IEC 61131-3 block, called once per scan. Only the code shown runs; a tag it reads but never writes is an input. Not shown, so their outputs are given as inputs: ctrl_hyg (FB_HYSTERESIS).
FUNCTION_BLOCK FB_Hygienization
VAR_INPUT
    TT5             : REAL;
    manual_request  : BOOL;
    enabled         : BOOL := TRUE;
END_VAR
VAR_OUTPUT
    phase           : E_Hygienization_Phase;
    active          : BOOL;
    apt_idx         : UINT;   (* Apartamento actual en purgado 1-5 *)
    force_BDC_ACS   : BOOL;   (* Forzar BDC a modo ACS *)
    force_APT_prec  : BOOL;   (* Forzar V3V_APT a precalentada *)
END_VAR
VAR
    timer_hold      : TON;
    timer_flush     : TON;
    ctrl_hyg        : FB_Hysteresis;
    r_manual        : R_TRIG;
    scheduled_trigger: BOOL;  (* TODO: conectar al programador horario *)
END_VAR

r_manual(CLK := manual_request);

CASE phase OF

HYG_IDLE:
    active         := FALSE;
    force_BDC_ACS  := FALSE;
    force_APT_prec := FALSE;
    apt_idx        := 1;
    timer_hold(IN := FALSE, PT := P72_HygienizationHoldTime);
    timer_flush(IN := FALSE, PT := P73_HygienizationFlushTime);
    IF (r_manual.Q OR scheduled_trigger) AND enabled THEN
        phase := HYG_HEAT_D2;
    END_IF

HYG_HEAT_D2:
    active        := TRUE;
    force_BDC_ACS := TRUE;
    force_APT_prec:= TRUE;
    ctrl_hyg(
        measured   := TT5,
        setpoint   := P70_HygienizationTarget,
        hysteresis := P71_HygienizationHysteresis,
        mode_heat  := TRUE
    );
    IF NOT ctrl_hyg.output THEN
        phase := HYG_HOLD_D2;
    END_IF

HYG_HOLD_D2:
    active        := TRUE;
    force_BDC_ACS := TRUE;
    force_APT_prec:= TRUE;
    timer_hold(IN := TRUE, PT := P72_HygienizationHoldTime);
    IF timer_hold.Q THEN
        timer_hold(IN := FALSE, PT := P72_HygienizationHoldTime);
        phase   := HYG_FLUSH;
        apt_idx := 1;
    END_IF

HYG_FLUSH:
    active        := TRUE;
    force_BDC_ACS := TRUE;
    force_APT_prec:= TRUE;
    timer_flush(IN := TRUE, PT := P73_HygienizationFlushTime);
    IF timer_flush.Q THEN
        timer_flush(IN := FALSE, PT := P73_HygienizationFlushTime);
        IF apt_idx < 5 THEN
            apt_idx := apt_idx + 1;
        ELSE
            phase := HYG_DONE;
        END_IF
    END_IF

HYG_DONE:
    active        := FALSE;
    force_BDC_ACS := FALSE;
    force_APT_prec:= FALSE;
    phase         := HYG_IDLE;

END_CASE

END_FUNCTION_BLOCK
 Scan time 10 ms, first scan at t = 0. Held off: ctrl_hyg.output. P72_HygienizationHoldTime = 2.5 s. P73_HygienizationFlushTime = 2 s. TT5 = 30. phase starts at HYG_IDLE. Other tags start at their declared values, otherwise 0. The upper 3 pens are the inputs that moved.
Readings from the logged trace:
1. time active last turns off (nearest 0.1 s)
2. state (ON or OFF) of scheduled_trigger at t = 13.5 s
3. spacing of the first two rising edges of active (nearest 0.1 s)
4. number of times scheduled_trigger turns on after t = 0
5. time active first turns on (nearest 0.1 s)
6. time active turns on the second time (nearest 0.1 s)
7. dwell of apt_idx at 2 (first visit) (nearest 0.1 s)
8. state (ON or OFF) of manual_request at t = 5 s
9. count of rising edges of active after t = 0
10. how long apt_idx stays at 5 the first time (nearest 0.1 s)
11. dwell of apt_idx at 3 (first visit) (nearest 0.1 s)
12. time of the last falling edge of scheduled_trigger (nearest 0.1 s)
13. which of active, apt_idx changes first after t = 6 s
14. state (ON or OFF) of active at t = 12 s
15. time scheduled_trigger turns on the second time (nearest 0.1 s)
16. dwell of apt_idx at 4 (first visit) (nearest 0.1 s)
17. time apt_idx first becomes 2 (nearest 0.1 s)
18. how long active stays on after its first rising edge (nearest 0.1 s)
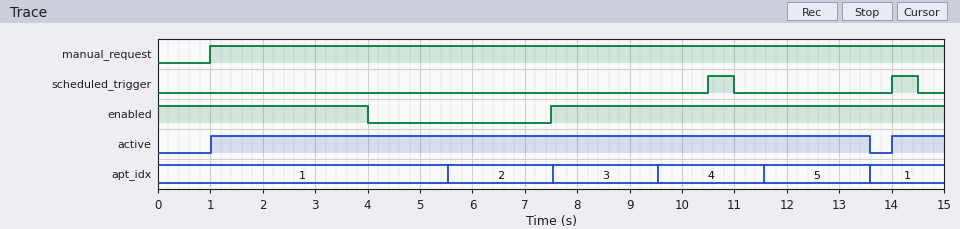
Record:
13.6 s
OFF
13.0 s
2
1.0 s
14.0 s
2.0 s
ON
2
2.0 s
2.0 s
14.5 s
apt_idx
ON
14.0 s
2.0 s
5.5 s
12.6 s
